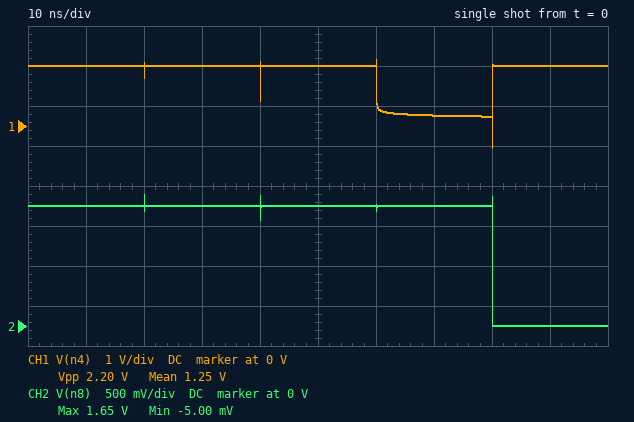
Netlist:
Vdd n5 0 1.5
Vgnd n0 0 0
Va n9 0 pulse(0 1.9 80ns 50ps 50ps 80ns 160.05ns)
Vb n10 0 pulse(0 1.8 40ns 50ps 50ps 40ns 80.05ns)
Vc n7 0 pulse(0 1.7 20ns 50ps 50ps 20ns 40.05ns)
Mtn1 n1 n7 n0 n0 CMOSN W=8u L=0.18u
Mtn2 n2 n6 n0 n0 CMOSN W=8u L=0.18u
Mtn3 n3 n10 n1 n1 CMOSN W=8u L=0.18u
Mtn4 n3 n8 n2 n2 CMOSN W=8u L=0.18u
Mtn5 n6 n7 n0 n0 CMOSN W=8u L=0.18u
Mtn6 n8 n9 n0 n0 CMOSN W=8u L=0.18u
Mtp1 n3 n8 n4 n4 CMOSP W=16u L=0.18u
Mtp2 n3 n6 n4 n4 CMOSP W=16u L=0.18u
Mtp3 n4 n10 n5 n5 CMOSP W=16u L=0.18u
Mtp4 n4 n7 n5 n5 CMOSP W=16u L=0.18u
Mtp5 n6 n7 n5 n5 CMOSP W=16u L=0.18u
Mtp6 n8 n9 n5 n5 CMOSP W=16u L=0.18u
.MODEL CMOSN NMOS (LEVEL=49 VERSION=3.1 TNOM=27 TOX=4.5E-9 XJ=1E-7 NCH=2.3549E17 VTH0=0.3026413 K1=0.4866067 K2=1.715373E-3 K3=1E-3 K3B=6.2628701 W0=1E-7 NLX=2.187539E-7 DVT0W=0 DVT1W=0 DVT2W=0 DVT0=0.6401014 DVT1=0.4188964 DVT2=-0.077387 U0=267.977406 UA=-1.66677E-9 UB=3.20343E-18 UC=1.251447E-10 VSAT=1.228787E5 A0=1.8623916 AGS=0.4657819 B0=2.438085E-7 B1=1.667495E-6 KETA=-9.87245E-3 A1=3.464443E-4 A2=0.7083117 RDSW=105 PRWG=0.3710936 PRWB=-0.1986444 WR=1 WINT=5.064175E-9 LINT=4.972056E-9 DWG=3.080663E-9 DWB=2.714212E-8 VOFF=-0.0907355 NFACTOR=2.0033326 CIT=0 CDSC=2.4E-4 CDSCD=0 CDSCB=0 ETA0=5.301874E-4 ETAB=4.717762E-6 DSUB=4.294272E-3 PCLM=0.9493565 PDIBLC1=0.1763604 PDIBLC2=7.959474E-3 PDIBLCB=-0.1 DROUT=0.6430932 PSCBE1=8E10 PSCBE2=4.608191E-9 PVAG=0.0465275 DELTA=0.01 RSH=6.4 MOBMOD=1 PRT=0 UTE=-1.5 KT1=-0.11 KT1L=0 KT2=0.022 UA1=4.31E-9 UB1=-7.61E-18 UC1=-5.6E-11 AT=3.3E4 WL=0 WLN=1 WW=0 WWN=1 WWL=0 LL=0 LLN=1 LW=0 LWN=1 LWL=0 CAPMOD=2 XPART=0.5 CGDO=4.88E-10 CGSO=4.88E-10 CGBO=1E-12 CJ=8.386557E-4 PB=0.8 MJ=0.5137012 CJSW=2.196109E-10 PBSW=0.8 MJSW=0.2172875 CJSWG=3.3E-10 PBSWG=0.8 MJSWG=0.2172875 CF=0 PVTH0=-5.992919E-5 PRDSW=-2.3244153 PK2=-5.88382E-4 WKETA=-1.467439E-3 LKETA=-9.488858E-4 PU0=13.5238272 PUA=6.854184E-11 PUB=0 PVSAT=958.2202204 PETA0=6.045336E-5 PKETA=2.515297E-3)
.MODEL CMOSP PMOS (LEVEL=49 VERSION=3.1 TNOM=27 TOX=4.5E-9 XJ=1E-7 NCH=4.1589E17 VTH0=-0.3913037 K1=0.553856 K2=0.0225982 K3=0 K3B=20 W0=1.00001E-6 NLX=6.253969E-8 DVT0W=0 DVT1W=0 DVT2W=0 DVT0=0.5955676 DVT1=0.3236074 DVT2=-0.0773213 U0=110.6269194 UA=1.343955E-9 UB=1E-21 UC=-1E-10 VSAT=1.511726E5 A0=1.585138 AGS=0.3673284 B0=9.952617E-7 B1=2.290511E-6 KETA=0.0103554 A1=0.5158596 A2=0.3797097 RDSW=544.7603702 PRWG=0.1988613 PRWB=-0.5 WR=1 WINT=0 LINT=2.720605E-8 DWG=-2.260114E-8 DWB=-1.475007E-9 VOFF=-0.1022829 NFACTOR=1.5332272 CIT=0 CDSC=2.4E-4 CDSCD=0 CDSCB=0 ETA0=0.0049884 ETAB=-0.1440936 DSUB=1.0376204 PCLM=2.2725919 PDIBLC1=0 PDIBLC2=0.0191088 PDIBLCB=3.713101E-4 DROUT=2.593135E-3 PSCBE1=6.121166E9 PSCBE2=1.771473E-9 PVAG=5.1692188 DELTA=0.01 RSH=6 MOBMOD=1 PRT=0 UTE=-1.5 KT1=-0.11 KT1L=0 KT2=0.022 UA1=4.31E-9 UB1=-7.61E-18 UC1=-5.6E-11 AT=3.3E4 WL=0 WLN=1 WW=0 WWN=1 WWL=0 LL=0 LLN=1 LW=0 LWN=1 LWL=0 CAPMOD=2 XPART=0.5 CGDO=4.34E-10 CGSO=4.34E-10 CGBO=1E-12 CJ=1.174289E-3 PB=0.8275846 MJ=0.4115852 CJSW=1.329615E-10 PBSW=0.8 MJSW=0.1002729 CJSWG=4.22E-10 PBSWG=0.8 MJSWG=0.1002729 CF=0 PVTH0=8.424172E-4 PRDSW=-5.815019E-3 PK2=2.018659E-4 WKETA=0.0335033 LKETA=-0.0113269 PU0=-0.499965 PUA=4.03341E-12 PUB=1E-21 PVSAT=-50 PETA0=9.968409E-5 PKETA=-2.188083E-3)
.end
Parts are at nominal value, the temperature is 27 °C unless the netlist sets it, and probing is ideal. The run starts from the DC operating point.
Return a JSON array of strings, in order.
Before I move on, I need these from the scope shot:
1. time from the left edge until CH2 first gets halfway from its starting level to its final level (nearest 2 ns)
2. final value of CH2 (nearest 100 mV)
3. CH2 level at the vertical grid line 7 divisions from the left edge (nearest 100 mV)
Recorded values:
["80 ns", "0 V", "1.5 V"]
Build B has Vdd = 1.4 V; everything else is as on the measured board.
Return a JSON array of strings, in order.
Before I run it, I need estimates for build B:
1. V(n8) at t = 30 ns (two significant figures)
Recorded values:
["1.4 V"]
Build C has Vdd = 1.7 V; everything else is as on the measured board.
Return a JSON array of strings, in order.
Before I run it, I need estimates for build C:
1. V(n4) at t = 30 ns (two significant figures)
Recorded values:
["1.7 V"]
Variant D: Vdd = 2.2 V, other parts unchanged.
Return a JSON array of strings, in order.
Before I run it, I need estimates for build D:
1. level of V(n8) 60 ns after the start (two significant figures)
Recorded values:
["2.2 V"]
